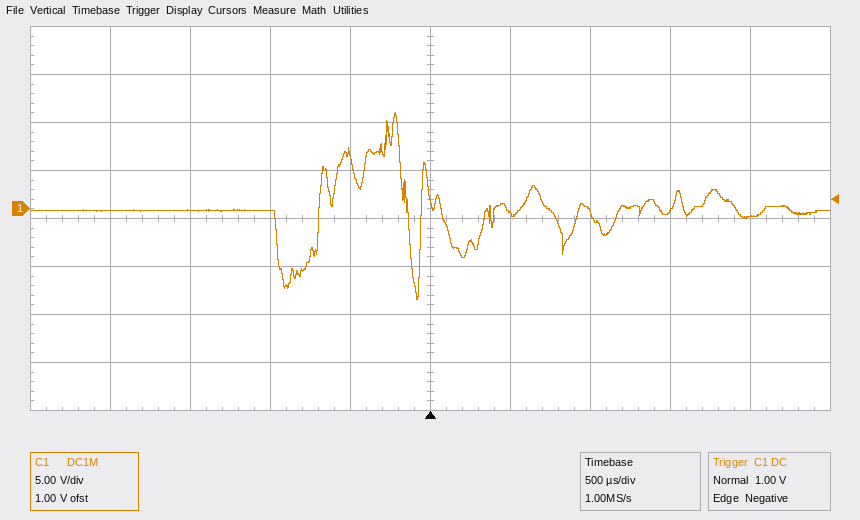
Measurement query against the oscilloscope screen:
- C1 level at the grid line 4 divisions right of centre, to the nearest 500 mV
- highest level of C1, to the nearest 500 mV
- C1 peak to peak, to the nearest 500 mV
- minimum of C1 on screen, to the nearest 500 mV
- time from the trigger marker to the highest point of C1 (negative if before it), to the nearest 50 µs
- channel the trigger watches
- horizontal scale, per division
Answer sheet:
-1.0 V
10.0 V
19.5 V
-9.5 V
-200 µs
C1
500 µs
